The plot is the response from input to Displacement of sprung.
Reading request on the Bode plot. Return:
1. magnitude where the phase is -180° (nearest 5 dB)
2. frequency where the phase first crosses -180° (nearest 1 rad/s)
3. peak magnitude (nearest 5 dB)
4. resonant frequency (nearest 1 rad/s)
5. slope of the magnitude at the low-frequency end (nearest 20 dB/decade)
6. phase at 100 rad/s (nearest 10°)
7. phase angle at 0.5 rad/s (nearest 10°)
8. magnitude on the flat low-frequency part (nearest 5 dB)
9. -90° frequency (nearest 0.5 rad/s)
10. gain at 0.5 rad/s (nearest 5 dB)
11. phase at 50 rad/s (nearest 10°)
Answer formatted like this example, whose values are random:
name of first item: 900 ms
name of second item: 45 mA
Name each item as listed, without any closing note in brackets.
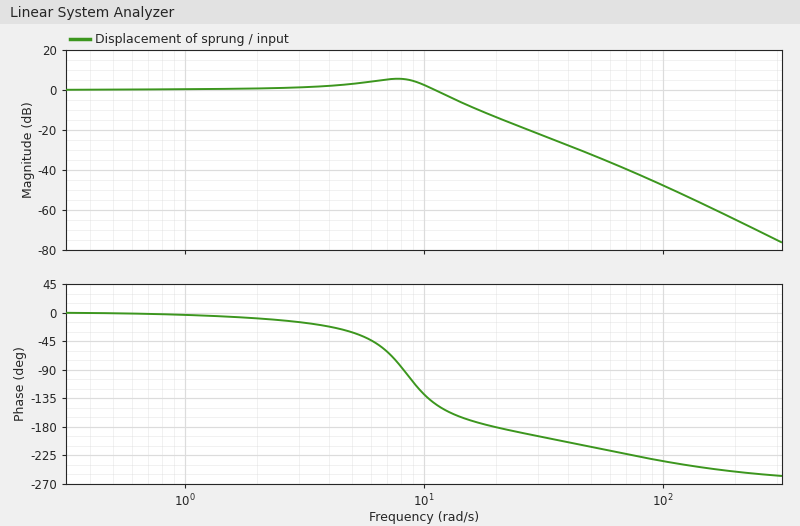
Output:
magnitude where the phase is -180°: -15 dB
frequency where the phase first crosses -180°: 20 rad/s
peak magnitude: 5 dB
resonant frequency: 8 rad/s
slope of the magnitude at the low-frequency end: 0 dB/decade
phase at 100 rad/s: -230°
phase angle at 0.5 rad/s: 0°
magnitude on the flat low-frequency part: 0 dB
-90° frequency: 8.0 rad/s
gain at 0.5 rad/s: 0 dB
phase at 50 rad/s: -210°
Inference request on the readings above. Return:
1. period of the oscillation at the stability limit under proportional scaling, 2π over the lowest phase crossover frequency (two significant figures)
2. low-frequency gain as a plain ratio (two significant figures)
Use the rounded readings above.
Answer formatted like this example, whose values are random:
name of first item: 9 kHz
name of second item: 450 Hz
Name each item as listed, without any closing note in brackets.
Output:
period of the oscillation at the stability limit under proportional scaling, 2π over the lowest phase crossover frequency: 0.31 s
low-frequency gain as a plain ratio: 1.0
